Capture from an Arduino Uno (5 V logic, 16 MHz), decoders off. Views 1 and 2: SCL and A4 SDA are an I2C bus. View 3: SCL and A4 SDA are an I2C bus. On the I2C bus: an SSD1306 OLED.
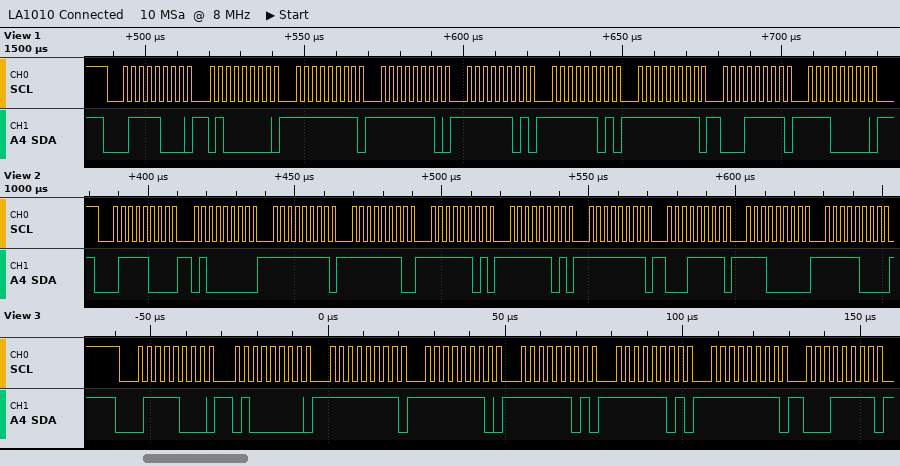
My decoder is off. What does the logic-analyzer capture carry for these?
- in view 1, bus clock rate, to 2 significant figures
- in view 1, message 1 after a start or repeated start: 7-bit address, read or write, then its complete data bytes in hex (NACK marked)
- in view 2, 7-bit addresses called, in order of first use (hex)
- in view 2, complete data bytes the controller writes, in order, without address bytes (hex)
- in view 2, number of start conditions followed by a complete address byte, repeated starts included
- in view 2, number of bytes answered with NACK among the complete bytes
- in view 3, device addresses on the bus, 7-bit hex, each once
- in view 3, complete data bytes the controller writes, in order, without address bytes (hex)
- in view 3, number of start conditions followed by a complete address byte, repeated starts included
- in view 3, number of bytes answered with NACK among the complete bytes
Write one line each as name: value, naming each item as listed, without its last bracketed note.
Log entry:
in view 1, bus clock rate, to 2 significant figures: 400 kHz
in view 1, message 1 after a start or repeated start: 7-bit address, read or write, then its complete data bytes in hex: 0x3C write: 40 FF FE FD FD FF 1F E0
in view 2, 7-bit addresses called, in order of first use: 0x3C
in view 2, complete data bytes the controller writes, in order, without address bytes: 40 FF FE FD FD FF 1F E0 F8
in view 2, number of start conditions followed by a complete address byte, repeated starts included: 1
in view 2, number of bytes answered with NACK among the complete bytes: 0
in view 3, device addresses on the bus, 7-bit hex, each once: 0x3C
in view 3, complete data bytes the controller writes, in order, without address bytes: 40 FF FE FD FD FF 1F
in view 3, number of start conditions followed by a complete address byte, repeated starts included: 1
in view 3, number of bytes answered with NACK among the complete bytes: 0
